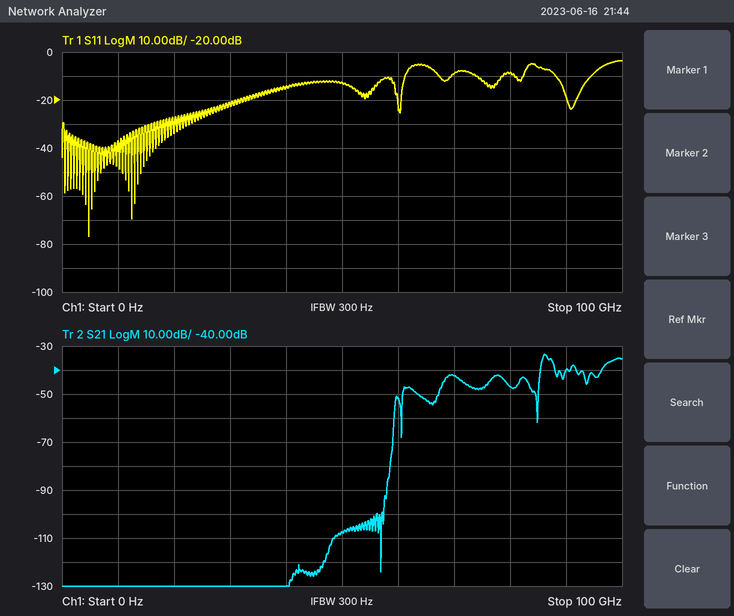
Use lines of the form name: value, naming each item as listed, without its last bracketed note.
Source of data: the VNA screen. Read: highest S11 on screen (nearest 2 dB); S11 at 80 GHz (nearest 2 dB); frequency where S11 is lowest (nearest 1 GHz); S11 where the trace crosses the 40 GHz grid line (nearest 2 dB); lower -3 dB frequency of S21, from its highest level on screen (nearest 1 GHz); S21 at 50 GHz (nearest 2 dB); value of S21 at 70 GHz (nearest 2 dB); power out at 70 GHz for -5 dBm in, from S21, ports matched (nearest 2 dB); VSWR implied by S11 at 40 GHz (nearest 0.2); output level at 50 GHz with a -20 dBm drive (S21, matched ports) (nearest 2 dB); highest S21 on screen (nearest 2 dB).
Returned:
highest S11 on screen: -4 dB
S11 at 80 GHz: -8 dB
frequency where S11 is lowest: 5 GHz
S11 where the trace crosses the 40 GHz grid line: -14 dB
lower -3 dB frequency of S21, from its highest level on screen: 86 GHz
S21 at 50 GHz: -108 dB
value of S21 at 70 GHz: -42 dB
power out at 70 GHz for -5 dBm in, from S21, ports matched: -48 dBm
VSWR implied by S11 at 40 GHz: 1.4
output level at 50 GHz with a -20 dBm drive (S21, matched ports): -128 dBm
highest S21 on screen: -34 dB
